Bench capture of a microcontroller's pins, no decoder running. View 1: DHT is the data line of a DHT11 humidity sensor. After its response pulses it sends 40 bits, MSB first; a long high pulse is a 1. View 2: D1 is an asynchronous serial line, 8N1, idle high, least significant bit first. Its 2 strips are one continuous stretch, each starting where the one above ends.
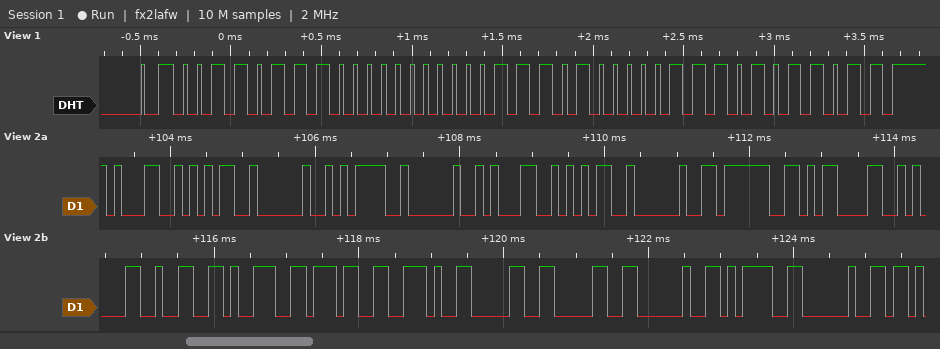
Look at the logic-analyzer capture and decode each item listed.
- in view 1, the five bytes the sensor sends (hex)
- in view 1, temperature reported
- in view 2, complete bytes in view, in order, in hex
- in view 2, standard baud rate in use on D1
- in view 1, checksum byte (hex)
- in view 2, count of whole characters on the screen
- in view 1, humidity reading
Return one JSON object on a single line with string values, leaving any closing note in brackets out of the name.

{"in view 1, the five bytes the sensor sends": "37 00 1D 07 5B", "in view 1, temperature reported": "29.7 °C", "in view 2, complete bytes in view, in order, in hex": "31 35 20 3D 20 31 35 20 3F 0D 0A 32 39 37 2E 30 30 20 3D 20", "in view 2, standard baud rate in use on D1": "9600 baud", "in view 1, checksum byte": "0x5B", "in view 2, count of whole characters on the screen": "20", "in view 1, humidity reading": "55 %"}
